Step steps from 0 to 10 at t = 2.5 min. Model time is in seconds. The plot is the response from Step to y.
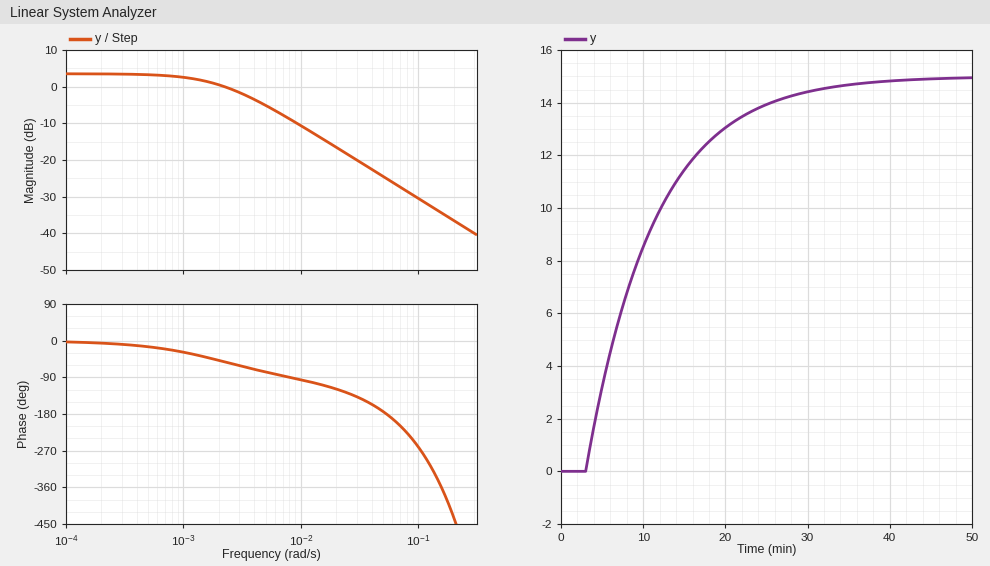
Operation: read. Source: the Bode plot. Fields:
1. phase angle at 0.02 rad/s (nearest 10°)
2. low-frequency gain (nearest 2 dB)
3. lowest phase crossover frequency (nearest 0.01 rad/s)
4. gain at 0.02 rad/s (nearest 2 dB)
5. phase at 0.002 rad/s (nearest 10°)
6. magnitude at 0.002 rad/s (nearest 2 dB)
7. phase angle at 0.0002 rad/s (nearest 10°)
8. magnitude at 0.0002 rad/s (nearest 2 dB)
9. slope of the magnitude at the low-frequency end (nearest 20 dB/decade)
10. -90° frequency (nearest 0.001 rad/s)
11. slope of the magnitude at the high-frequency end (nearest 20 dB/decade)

-120°
4 dB
0.05 rad/s
-16 dB
-50°
0 dB
-10°
4 dB
0 dB/decade
0.008 rad/s
-20 dB/decade
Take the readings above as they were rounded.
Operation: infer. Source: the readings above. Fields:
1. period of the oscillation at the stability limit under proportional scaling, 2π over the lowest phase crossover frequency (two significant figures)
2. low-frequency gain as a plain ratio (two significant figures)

130 s
1.6
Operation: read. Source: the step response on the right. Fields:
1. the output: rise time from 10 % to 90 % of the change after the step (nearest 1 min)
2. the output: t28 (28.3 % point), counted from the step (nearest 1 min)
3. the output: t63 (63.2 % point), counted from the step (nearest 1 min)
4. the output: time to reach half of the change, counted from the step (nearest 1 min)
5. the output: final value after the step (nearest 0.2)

18 min
3 min
9 min
6 min
15.0
